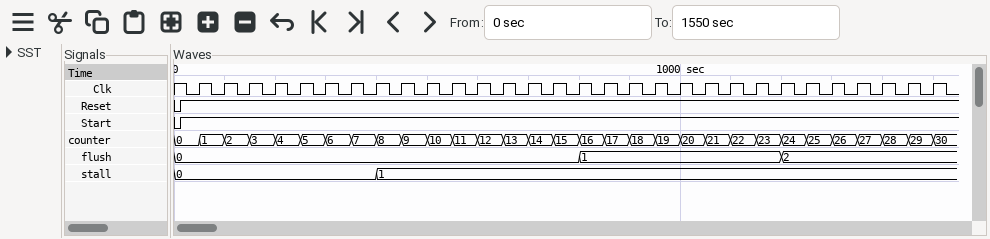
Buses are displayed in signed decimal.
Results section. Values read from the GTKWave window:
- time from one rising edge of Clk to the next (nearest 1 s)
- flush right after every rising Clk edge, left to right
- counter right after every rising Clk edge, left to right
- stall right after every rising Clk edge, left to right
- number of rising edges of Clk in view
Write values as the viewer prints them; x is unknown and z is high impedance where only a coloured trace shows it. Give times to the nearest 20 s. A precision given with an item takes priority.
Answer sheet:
50 s
0, 0, 0, 0, 0, 0, 0, 0, 0, 0, 0, 0, 0, 0, 0, 1, 1, 1, 1, 1, 1, 1, 1, 2, 2, 2, 2, 2, 2, 2
1, 2, 3, 4, 5, 6, 7, 8, 9, 10, 11, 12, 13, 14, 15, 16, 17, 18, 19, 20, 21, 22, 23, 24, 25, 26, 27, 28, 29, 30
0, 0, 0, 0, 0, 0, 0, 1, 1, 1, 1, 1, 1, 1, 1, 1, 1, 1, 1, 1, 1, 1, 1, 1, 1, 1, 1, 1, 1, 1
30
